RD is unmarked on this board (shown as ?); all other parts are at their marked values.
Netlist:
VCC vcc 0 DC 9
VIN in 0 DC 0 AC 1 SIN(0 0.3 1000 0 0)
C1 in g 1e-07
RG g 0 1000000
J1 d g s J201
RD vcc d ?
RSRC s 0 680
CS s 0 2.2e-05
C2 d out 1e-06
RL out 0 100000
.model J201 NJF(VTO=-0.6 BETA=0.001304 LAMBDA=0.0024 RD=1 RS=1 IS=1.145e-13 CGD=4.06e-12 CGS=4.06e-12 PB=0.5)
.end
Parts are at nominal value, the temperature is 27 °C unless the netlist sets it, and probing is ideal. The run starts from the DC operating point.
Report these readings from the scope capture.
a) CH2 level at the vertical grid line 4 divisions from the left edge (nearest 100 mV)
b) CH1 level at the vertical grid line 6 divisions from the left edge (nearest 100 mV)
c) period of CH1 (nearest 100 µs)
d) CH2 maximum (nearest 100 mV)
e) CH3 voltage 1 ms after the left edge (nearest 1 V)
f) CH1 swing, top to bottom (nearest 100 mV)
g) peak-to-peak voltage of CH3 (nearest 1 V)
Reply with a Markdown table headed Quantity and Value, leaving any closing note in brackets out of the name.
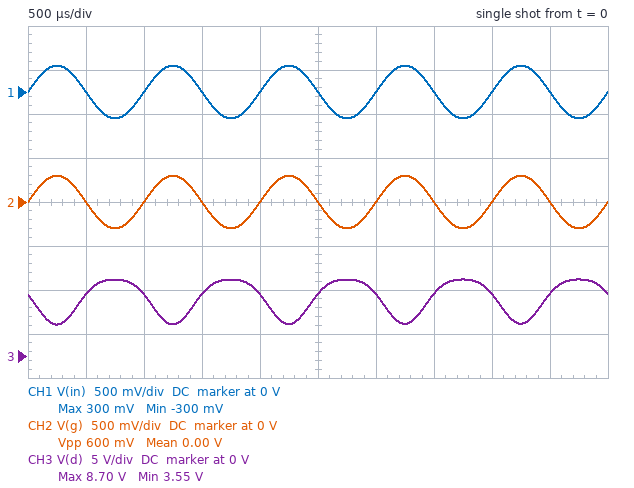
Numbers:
| Quantity | Value |
|---|---|
| CH2 level at the vertical grid line 4 divisions from the left edge | 0 V |
| CH1 level at the vertical grid line 6 divisions from the left edge | 0 V |
| period of CH1 | 1.0 ms |
| CH2 maximum | 300 mV |
| CH3 voltage 1 ms after the left edge | 7 V |
| CH1 swing, top to bottom | 600 mV |
| peak-to-peak voltage of CH3 | 5 V |
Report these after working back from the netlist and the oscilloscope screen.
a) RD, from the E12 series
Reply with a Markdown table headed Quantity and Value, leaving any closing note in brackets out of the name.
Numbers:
| Quantity | Value |
|---|---|
| RD, from the E12 series | 8.2 kΩ |
